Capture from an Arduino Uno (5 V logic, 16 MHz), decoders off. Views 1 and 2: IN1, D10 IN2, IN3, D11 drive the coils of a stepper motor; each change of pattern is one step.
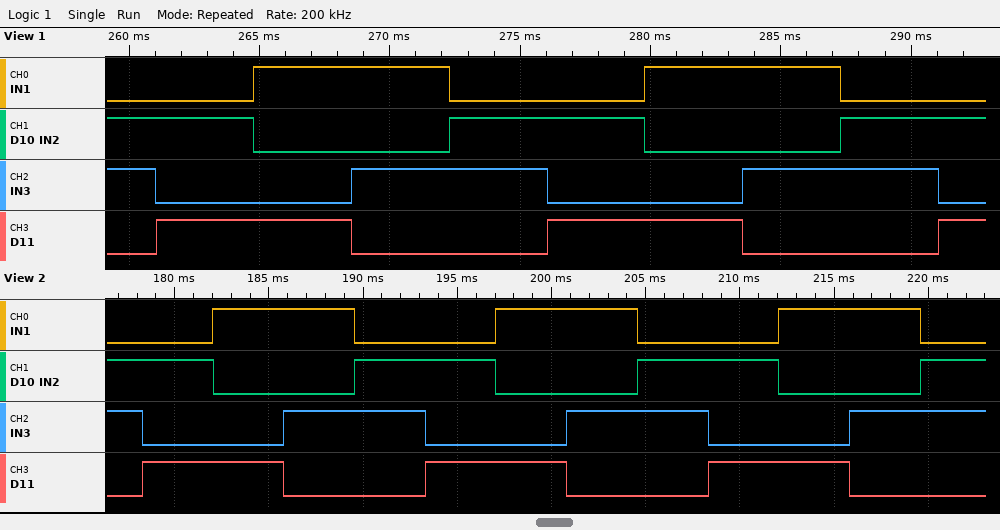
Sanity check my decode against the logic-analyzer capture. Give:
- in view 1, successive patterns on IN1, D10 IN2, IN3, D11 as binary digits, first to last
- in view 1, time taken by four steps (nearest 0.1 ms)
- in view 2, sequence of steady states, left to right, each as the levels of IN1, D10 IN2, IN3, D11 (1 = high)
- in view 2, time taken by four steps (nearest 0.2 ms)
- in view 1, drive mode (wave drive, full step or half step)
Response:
0110 0101 1001 1010 0110 0101 1001 1010 0110 0101
15.0 ms
0110 0101 1001 1010 0110 0101 1001 1010 0110 0101 1001 1010 0110
15.0 ms
full step
